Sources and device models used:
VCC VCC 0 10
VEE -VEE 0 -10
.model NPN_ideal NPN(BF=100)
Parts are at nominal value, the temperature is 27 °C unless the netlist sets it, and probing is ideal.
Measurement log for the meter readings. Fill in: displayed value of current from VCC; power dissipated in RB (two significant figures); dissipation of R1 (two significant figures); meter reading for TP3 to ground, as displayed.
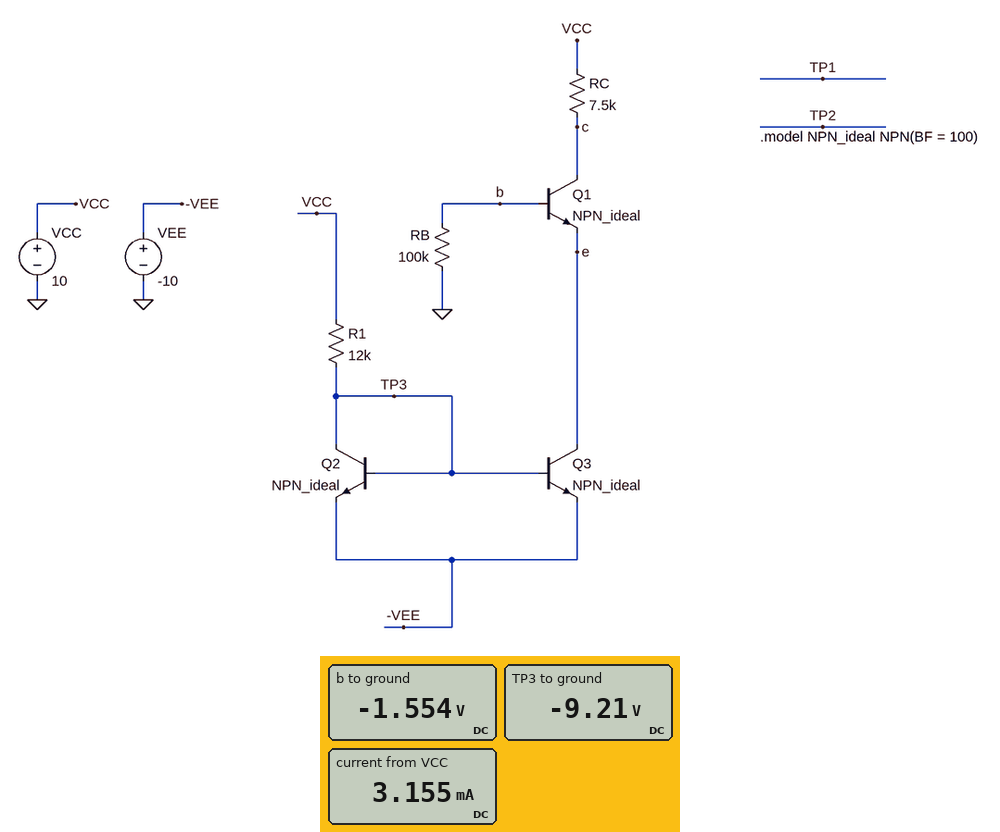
3.155 mA
24 µW
31 mW
-9.21 V
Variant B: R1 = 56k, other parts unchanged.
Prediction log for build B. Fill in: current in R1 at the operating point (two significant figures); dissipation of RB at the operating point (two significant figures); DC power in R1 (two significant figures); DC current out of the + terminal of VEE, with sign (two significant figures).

340 µA
1.1 µW
6.6 mW
-680 µA
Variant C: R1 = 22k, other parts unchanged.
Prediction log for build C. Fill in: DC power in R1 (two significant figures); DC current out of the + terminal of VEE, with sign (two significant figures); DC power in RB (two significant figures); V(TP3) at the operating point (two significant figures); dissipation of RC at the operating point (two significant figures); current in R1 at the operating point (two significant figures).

17 mW
-1.7 mA
7.2 µW
-9.2 V
5.4 mW
870 µA
